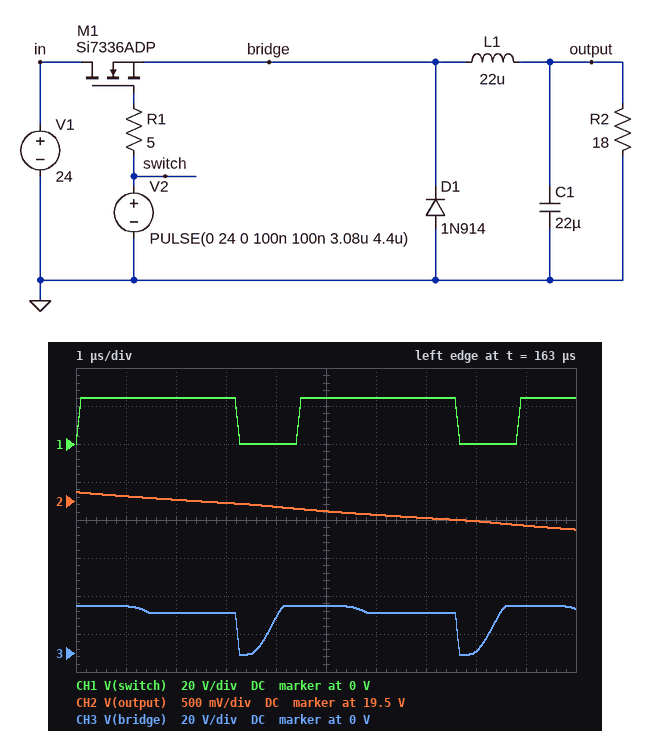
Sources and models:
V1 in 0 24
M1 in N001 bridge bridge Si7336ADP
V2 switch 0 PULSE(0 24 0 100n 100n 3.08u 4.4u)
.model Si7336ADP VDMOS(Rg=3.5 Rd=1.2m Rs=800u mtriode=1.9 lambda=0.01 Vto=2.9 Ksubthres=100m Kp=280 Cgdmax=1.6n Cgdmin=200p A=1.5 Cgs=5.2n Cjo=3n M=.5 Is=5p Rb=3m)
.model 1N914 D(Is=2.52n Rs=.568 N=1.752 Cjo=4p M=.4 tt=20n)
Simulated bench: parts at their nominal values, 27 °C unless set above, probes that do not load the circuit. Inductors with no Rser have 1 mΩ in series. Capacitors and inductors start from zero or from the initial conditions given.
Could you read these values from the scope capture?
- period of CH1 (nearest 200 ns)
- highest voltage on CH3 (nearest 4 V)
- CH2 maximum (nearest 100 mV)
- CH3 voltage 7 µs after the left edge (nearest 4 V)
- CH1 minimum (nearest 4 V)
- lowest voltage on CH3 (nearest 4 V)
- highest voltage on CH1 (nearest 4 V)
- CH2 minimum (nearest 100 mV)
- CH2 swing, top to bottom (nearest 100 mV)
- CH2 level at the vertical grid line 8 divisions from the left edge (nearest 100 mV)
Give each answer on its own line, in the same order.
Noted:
4.4 µs
24 V
19.6 V
20 V
0 V
0 V
24 V
19.1 V
500 mV
19.2 V
